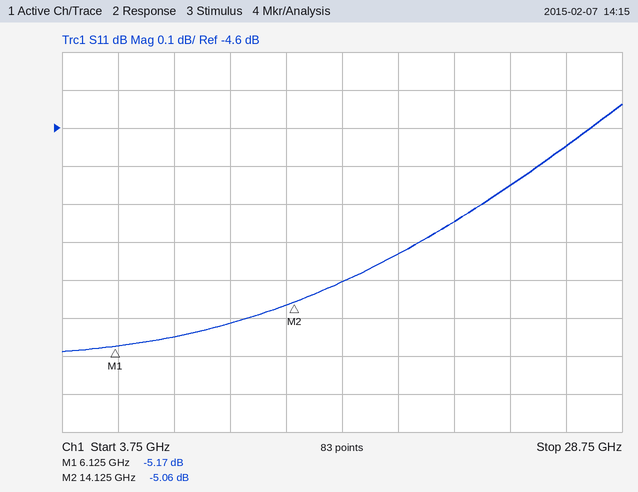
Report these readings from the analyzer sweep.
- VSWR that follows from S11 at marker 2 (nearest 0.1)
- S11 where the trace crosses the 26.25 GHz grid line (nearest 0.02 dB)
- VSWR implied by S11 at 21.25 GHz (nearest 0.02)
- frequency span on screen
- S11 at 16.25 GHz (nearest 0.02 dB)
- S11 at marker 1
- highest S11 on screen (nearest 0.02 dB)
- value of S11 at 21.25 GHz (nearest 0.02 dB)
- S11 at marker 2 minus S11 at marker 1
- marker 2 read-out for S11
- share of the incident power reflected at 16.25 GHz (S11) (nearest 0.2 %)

3.5
-4.64 dB
3.68
25 GHz
-5.00 dB
-5.17 dB
-4.54 dB
-4.84 dB
0.11 dB
-5.06 dB
31.6 %
